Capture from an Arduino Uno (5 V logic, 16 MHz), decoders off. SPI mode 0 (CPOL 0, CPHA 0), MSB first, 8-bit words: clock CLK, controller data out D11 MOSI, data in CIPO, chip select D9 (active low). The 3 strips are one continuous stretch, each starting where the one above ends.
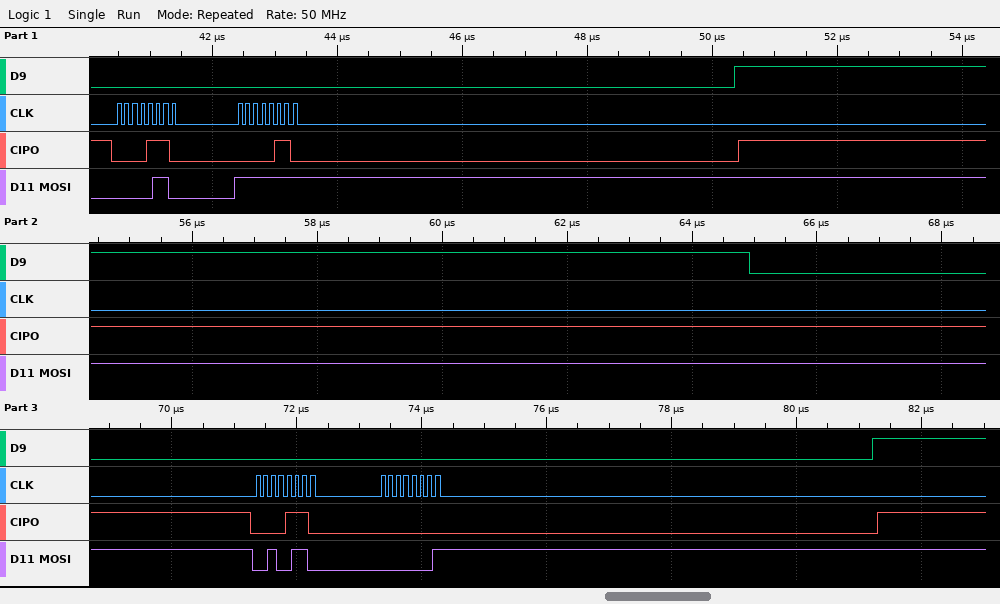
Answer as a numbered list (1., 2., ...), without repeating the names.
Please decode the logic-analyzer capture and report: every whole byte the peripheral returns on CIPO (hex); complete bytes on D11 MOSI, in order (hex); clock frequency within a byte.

1. 0E 06 0E 00
2. 06 FF 26 01
3. 8 MHz
